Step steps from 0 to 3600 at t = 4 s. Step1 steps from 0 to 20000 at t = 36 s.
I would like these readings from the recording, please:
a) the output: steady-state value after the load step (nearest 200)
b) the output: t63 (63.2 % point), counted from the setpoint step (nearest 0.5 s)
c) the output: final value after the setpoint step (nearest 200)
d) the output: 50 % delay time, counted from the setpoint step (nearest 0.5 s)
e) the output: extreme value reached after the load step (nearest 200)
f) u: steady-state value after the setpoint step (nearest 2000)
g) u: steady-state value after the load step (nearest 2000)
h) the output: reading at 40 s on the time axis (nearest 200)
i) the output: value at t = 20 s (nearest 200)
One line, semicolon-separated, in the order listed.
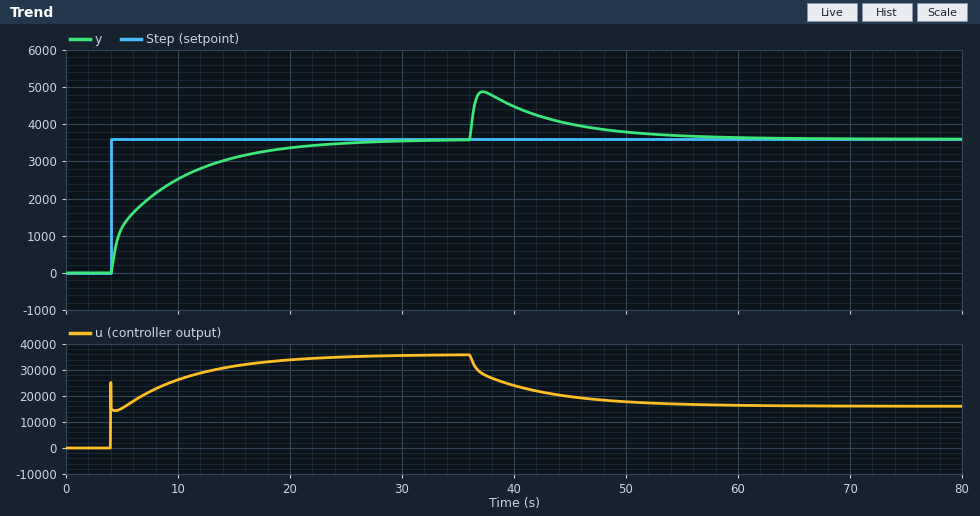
3600; 4.5 s; 3600; 2.5 s; 4800; 36000; 16000; 4400; 3400
